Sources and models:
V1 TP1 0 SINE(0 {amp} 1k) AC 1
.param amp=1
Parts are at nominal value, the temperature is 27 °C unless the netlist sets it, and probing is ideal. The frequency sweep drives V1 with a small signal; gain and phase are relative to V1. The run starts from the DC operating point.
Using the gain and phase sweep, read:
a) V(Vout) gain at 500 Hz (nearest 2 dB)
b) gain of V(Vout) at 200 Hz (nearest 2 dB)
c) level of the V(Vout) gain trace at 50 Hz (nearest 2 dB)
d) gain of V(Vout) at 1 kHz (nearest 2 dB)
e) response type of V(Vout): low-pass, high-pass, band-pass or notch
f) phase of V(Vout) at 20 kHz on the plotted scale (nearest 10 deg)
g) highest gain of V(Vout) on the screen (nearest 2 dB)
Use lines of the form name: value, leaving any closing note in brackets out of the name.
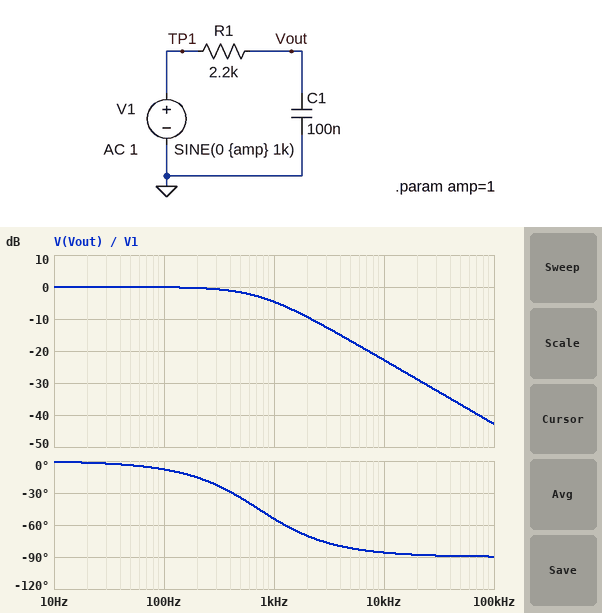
V(Vout) gain at 500 Hz: -2 dB
gain of V(Vout) at 200 Hz: 0 dB
level of the V(Vout) gain trace at 50 Hz: 0 dB
gain of V(Vout) at 1 kHz: -4 dB
response type of V(Vout): low-pass, high-pass, band-pass or notch: low-pass
phase of V(Vout) at 20 kHz on the plotted scale: -90 deg
highest gain of V(Vout) on the screen: 0 dB
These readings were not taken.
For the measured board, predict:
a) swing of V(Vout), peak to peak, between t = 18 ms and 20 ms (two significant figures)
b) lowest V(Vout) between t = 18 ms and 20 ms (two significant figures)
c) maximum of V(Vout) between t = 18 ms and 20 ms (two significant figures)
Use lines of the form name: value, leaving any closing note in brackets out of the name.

swing of V(Vout), peak to peak, between t = 18 ms and 20 ms: 1.2 V
lowest V(Vout) between t = 18 ms and 20 ms: -590 mV
maximum of V(Vout) between t = 18 ms and 20 ms: 590 mV
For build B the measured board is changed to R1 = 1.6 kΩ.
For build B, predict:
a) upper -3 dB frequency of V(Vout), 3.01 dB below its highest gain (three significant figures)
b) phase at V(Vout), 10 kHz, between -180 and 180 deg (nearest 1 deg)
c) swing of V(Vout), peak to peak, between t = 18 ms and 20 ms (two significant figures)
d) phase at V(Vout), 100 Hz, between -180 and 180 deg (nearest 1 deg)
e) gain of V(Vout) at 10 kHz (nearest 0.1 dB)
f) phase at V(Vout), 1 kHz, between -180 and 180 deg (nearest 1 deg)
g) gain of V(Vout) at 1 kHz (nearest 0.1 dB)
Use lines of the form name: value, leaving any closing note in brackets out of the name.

upper -3 dB frequency of V(Vout), 3.01 dB below its highest gain: 995 Hz
phase at V(Vout), 10 kHz, between -180 and 180 deg: -84 deg
swing of V(Vout), peak to peak, between t = 18 ms and 20 ms: 1.4 V
phase at V(Vout), 100 Hz, between -180 and 180 deg: -6 deg
gain of V(Vout) at 10 kHz: -20.1 dB
phase at V(Vout), 1 kHz, between -180 and 180 deg: -45 deg
gain of V(Vout) at 1 kHz: -3.0 dB
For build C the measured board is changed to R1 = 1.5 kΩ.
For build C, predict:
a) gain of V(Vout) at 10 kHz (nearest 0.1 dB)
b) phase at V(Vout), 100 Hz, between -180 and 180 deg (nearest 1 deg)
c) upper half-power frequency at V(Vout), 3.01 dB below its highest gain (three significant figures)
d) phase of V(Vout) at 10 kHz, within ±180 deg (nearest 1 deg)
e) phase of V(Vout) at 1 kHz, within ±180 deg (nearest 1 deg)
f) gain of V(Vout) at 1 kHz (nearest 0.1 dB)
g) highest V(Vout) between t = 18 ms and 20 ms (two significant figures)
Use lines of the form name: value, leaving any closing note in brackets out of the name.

gain of V(Vout) at 10 kHz: -19.5 dB
phase at V(Vout), 100 Hz, between -180 and 180 deg: -5 deg
upper half-power frequency at V(Vout), 3.01 dB below its highest gain: 1.06 kHz
phase of V(Vout) at 10 kHz, within ±180 deg: -84 deg
phase of V(Vout) at 1 kHz, within ±180 deg: -43 deg
gain of V(Vout) at 1 kHz: -2.8 dB
highest V(Vout) between t = 18 ms and 20 ms: 730 mV
